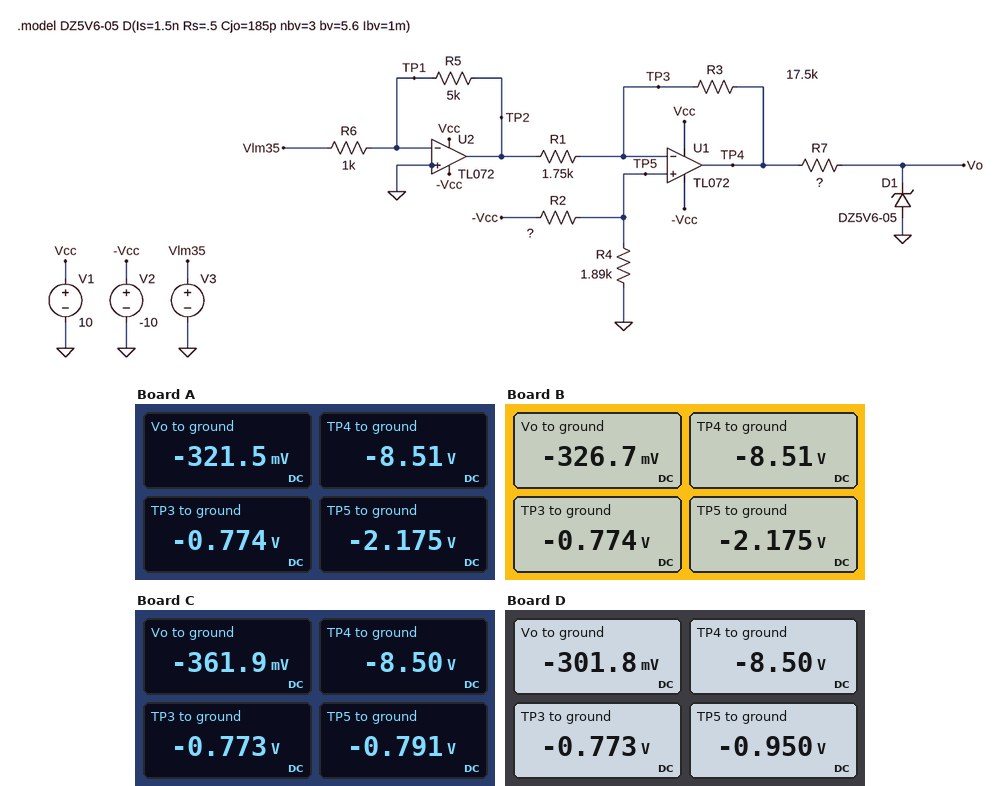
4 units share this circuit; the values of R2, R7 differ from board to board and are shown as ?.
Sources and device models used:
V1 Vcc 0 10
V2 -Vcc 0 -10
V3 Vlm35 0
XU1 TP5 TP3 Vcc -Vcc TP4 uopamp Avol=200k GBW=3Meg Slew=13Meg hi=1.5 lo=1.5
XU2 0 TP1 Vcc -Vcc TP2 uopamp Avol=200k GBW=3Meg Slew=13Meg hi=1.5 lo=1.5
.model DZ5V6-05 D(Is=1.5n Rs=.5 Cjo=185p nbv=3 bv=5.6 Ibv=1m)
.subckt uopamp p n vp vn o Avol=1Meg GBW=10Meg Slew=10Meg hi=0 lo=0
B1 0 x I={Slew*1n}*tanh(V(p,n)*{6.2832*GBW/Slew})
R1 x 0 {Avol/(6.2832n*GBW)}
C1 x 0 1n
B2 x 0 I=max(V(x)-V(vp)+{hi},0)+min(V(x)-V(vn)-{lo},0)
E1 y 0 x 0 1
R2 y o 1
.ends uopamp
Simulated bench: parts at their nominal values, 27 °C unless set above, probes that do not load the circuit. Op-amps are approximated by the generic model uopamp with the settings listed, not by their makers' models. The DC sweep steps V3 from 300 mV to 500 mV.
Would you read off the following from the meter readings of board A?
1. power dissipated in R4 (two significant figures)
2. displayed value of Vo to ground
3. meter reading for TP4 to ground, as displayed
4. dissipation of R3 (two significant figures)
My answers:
2.5 mW
-321.5 mV
-8.51 V
3.4 mW
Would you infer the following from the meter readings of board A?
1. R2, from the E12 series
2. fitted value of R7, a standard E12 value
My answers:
6.8 kΩ
22 kΩ
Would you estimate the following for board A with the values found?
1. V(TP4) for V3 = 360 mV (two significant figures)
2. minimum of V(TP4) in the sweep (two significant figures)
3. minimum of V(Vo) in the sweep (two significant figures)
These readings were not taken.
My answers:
-5.9 V
-8.5 V
-320 mV
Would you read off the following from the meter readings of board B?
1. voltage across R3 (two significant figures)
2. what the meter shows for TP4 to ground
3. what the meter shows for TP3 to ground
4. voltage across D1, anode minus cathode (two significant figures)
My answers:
7.7 V
-8.51 V
-0.774 V
330 mV
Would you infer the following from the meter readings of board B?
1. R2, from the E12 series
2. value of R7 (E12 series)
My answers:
6.8 kΩ
18 kΩ
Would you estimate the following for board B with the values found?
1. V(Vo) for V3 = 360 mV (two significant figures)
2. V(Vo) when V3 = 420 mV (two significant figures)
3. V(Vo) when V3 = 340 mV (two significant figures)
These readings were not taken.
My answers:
-320 mV
-300 mV
-320 mV
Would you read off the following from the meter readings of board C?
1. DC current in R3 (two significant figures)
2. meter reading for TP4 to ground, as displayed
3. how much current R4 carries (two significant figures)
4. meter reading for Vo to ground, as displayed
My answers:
440 µA
-8.50 V
420 µA
-361.9 mV
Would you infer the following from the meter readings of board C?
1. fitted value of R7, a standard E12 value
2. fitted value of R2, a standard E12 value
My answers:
4.7 kΩ
22 kΩ
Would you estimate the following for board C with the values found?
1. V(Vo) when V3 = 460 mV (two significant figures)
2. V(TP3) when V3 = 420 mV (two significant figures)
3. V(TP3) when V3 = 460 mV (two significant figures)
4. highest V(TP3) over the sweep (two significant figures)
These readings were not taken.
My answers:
5.6 V
-1.1 V
-1.3 V
-790 mV
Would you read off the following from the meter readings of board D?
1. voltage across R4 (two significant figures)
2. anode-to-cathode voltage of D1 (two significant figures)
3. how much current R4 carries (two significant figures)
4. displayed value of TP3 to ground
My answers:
950 mV
300 mV
500 µA
-0.773 V
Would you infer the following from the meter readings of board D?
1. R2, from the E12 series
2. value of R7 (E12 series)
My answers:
18 kΩ
47 kΩ
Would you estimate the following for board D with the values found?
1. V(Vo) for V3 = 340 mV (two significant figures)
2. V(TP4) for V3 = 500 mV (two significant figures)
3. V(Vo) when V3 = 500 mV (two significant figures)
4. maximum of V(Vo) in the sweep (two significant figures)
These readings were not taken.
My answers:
5.3 V
8.5 V
5.4 V
5.4 V
